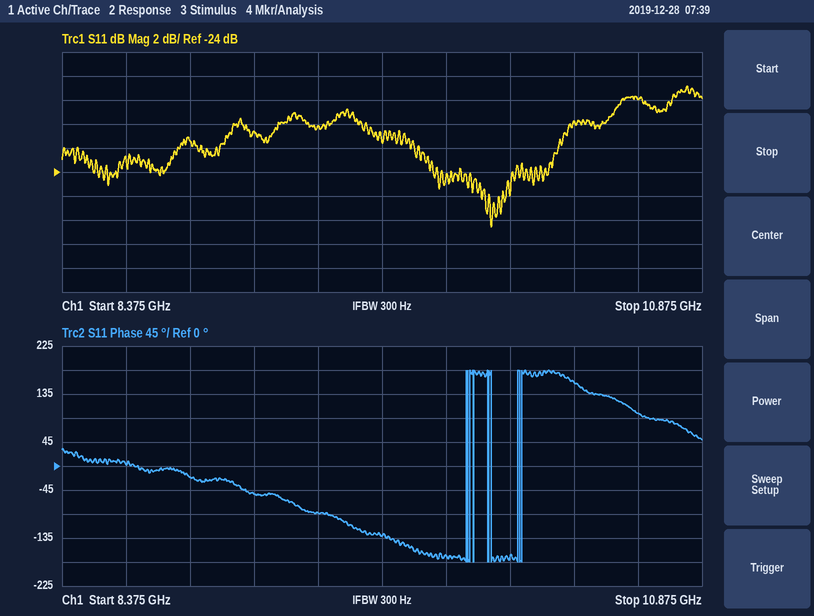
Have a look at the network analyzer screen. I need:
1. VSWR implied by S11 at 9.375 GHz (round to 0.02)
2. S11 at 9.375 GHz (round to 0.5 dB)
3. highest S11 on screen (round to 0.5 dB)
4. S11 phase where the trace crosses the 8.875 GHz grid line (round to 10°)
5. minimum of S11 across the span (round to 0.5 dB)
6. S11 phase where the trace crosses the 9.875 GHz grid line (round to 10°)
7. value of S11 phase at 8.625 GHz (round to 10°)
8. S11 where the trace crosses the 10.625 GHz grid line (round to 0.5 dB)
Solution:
1.22
-20.0 dB
-17.0 dB
-20°
-28.5 dB
-170°
0°
-18.0 dB
